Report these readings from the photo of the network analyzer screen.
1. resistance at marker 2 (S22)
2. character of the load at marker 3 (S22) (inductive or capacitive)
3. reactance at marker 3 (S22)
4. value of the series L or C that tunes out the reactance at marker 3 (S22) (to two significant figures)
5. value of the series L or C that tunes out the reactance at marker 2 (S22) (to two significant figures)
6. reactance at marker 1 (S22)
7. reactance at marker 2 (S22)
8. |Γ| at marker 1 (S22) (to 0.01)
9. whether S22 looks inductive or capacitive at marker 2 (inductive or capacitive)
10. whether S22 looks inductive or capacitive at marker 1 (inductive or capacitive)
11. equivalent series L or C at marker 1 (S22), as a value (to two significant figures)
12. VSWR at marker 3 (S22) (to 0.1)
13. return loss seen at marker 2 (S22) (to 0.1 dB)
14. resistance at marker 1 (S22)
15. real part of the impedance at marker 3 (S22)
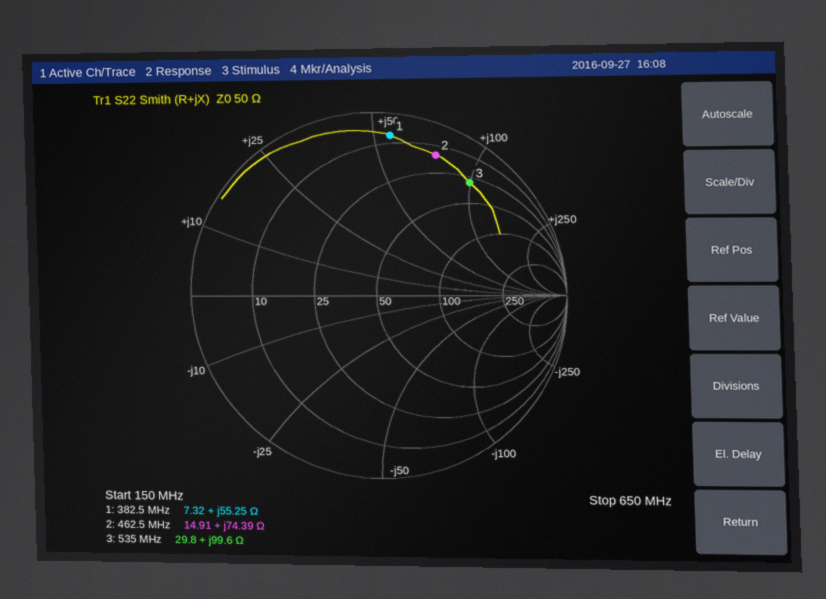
14.91 Ω
inductive
+99.6 Ω
3.0 pF
4.6 pF
+55.25 Ω
+74.39 Ω
0.88
inductive
inductive
23 nH
8.8
1.6 dB
7.32 Ω
29.8 Ω
